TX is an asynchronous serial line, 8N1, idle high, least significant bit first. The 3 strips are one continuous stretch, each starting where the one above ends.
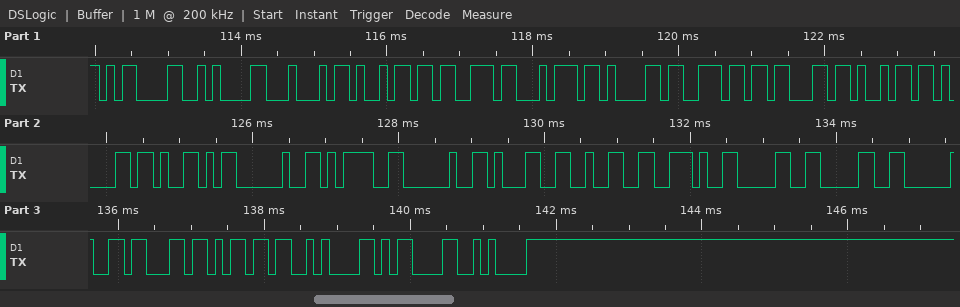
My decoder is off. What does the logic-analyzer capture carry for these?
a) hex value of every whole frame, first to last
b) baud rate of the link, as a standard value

0x0D 0x0A 0x44 0x69 0x73 0x74 0x61 0x6E 0x63 0x69 0x61 0x59 0x20 0x3D 0x20 0x31 0x32 0x2E 0x30 0x30 0x20 0x63 0x6D 0x0A 0x0D 0x0A
9600 baud
